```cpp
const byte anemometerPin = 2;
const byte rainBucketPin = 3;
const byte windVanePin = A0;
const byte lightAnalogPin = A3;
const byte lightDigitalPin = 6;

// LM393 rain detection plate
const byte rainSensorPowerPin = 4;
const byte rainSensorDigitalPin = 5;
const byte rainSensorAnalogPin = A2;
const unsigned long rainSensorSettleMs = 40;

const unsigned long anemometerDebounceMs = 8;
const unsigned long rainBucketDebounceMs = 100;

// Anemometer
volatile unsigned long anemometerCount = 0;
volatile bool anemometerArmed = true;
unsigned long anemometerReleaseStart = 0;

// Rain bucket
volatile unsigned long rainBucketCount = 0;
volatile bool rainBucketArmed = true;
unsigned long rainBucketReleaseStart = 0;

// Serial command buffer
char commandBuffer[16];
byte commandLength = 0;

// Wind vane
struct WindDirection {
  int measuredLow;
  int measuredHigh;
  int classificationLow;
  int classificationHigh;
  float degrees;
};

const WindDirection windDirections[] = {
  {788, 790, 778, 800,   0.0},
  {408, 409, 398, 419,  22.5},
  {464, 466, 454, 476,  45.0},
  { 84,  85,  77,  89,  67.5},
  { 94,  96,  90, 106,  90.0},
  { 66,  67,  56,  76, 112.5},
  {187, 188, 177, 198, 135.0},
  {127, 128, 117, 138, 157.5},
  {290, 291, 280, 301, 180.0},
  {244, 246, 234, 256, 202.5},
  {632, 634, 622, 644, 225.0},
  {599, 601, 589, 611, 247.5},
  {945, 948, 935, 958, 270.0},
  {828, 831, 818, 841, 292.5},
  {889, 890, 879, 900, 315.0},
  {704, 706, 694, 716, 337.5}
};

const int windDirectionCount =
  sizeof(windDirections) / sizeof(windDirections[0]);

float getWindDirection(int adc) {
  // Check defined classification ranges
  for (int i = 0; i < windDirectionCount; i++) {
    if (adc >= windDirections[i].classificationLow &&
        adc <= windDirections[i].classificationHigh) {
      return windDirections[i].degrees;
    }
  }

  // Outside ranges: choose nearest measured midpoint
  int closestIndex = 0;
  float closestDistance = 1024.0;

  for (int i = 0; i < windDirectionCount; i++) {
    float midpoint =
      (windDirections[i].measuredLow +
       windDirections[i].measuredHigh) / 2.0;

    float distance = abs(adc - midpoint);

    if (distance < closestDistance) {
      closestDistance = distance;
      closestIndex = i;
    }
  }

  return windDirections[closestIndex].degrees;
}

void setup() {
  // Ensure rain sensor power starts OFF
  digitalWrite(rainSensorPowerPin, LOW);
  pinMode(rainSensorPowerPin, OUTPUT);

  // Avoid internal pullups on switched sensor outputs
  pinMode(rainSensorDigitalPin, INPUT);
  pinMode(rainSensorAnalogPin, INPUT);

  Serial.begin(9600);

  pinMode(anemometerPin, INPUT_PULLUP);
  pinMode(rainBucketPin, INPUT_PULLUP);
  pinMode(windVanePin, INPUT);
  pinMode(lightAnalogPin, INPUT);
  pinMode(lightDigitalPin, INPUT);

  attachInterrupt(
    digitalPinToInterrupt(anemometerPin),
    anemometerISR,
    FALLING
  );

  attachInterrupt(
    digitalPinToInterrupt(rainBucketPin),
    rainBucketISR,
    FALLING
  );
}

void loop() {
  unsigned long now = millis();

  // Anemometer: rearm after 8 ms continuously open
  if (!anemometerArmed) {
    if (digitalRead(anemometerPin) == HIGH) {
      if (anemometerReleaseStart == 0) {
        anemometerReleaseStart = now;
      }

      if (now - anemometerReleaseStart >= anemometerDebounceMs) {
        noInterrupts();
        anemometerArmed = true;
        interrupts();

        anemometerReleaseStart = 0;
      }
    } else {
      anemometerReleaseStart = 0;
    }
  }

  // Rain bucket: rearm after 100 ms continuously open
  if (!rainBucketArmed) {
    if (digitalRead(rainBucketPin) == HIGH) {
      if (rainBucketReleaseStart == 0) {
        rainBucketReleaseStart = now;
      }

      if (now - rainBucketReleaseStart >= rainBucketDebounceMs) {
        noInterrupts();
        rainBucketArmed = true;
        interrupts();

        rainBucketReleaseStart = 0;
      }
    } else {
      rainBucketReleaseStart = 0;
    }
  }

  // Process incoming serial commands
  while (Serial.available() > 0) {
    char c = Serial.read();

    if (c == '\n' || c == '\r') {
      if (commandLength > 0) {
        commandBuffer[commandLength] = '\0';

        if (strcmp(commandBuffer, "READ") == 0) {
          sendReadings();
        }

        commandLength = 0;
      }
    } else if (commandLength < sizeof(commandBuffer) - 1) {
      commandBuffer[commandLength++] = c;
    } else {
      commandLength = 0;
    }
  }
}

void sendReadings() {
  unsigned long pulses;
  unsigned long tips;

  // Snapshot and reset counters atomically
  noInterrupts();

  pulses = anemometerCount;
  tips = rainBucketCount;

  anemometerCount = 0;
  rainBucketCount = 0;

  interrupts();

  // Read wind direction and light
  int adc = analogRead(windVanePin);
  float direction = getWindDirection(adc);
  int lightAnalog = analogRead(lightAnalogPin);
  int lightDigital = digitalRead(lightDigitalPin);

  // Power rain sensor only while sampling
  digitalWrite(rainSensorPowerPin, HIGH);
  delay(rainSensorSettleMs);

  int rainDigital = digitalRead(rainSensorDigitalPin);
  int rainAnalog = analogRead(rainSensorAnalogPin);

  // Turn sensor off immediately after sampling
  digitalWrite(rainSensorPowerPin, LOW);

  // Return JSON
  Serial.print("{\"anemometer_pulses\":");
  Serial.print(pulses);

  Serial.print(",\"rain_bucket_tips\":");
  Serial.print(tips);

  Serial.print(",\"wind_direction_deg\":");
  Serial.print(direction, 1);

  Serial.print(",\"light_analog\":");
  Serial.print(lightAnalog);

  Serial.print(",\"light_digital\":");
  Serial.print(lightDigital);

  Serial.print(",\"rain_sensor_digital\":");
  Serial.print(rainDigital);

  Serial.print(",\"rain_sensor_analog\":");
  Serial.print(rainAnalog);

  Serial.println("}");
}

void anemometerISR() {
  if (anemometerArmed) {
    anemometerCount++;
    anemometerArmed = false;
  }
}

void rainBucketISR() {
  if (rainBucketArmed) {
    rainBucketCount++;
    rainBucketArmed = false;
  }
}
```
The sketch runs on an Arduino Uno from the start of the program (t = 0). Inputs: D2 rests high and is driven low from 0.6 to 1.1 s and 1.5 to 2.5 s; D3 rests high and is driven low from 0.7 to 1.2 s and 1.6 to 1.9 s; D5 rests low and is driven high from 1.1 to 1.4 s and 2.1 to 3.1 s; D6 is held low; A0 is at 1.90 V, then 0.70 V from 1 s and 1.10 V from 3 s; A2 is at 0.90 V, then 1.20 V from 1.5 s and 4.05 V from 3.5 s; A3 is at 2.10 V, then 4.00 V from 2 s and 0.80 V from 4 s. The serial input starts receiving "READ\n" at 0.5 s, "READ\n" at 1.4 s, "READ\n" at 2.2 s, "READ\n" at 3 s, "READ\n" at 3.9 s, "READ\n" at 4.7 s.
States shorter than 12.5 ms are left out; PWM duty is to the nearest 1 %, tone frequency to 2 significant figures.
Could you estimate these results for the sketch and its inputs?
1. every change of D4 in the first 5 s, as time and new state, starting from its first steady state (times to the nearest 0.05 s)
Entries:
0 s low; 0.5 s high; 0.55 s low; 1.4 s high; 1.45 s low; 2.2 s high; 2.25 s low; 3 s high; 3.05 s low; 3.9 s high; 3.95 s low; 4.7 s high; 4.75 s low
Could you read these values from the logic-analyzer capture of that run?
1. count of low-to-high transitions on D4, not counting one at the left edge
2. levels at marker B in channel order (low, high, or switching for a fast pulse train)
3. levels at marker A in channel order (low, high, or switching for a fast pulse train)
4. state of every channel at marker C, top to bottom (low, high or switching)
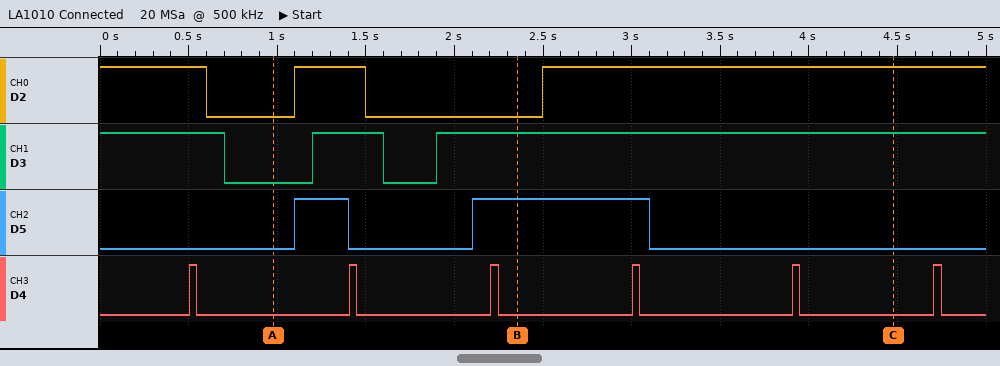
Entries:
6
D2 low, D3 high, D5 high, D4 low
D2 low, D3 low, D5 low, D4 low
D2 high, D3 high, D5 low, D4 low
